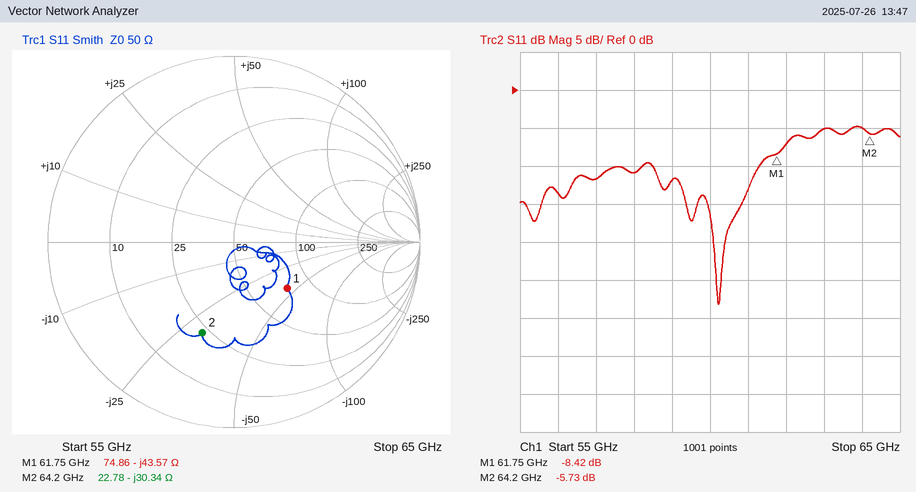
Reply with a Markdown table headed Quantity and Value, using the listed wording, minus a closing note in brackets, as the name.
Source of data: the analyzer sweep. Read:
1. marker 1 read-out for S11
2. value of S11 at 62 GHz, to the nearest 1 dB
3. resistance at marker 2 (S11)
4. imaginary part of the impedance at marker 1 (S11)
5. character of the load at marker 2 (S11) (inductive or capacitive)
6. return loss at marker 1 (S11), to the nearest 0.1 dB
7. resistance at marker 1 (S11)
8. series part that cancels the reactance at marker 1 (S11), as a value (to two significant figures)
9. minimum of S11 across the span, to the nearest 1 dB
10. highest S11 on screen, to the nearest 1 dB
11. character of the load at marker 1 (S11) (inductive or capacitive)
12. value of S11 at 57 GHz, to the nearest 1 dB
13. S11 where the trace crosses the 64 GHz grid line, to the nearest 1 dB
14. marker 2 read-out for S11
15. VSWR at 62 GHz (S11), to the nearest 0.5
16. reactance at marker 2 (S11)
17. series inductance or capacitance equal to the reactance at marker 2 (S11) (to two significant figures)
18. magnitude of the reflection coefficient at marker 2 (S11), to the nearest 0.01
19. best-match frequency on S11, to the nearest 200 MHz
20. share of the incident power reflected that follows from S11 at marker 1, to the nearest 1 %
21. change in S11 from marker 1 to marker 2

| Quantity | Value |
|---|---|
| marker 1 read-out for S11 | -8.42 dB |
| value of S11 at 62 GHz, to the nearest 1 dB | -7 dB |
| resistance at marker 2 | 22.78 Ω |
| imaginary part of the impedance at marker 1 | -43.57 Ω |
| character of the load at marker 2 (S11) | capacitive |
| return loss at marker 1 (S11), to the nearest 0.1 dB | 8.4 dB |
| resistance at marker 1 | 74.86 Ω |
| series part that cancels the reactance at marker 1 (S11), as a value | 110 pH |
| minimum of S11 across the span, to the nearest 1 dB | -28 dB |
| highest S11 on screen, to the nearest 1 dB | -5 dB |
| character of the load at marker 1 (S11) | capacitive |
| value of S11 at 57 GHz, to the nearest 1 dB | -12 dB |
| S11 where the trace crosses the 64 GHz grid line, to the nearest 1 dB | -5 dB |
| marker 2 read-out for S11 | -5.73 dB |
| VSWR at 62 GHz (S11), to the nearest 0.5 | 2.5 |
| reactance at marker 2 | -30.34 Ω |
| series inductance or capacitance equal to the reactance at marker 2 (S11) | 82 fF |
| magnitude of the reflection coefficient at marker 2 (S11), to the nearest 0.01 | 0.52 |
| best-match frequency on S11, to the nearest 200 MHz | 60.2 GHz |
| share of the incident power reflected that follows from S11 at marker 1, to the nearest 1 % | 14 % |
| change in S11 from marker 1 to marker 2 | 2.69 dB |
